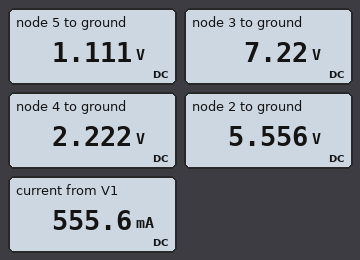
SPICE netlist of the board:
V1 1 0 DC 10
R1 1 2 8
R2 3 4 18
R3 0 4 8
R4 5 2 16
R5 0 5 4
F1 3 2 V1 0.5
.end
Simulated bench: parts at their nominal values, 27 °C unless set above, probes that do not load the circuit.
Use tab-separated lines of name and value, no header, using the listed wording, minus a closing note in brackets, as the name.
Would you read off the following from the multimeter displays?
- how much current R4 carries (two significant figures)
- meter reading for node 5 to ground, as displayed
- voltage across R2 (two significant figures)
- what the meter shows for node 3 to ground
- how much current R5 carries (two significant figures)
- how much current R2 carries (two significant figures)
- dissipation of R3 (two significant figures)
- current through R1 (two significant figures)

how much current R4 carries	280 mA
meter reading for node 5 to ground, as displayed	1.111 V
voltage across R2	5.0 V
what the meter shows for node 3 to ground	7.22 V
how much current R5 carries	280 mA
how much current R2 carries	280 mA
dissipation of R3	620 mW
current through R1	560 mA
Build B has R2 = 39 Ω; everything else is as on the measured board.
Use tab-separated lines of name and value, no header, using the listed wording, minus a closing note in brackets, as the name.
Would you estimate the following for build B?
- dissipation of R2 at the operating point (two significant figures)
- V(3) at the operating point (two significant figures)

dissipation of R2 at the operating point	3.0 W
V(3) at the operating point	13 V
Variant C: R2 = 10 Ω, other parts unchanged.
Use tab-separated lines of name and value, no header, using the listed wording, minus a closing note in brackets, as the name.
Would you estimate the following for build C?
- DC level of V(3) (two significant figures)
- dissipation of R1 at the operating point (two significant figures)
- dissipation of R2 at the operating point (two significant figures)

DC level of V(3)	5.0 V
dissipation of R1 at the operating point	2.5 W
dissipation of R2 at the operating point	770 mW
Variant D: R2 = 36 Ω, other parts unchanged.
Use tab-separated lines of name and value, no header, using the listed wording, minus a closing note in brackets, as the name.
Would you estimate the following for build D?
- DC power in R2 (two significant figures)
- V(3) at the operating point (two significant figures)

DC power in R2	2.8 W
V(3) at the operating point	12 V
